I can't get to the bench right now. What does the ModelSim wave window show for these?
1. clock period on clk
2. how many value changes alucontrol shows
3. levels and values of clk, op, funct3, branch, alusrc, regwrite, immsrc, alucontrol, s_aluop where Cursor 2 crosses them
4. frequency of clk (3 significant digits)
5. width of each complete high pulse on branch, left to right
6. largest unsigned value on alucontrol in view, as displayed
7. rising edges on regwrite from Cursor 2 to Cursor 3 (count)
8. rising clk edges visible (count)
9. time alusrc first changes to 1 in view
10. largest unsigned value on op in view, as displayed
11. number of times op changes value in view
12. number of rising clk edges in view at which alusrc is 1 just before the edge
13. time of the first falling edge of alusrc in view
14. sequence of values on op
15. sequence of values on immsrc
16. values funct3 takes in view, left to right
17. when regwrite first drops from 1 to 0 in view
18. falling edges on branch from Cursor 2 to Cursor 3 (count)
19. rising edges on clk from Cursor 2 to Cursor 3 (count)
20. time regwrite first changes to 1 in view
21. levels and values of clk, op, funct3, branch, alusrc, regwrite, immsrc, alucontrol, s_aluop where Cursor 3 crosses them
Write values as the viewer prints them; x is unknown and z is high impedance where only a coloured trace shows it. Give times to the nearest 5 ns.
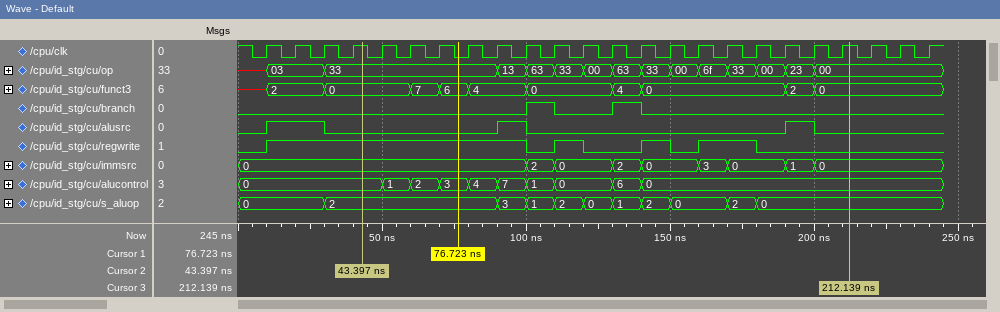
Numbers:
10 ns
9
clk=1, op=33, funct3=0, branch=0, alusrc=0, regwrite=1, immsrc=0, alucontrol=0, s_aluop=2
100 MHz
10 ns, 10 ns
7
3
24
10 ns
6f
14
4
30 ns
x, 03, 33, 13, 63, 33, 00, 63, 33, 00, 6f, 33, 00, 23, 00
0, 2, 0, 2, 0, 3, 0, 1, 0
x, 2, 0, 7, 6, 4, 0, 4, 0, 2, 0
100 ns
2
17
10 ns
clk=1, op=00, funct3=0, branch=0, alusrc=0, regwrite=0, immsrc=0, alucontrol=0, s_aluop=0
